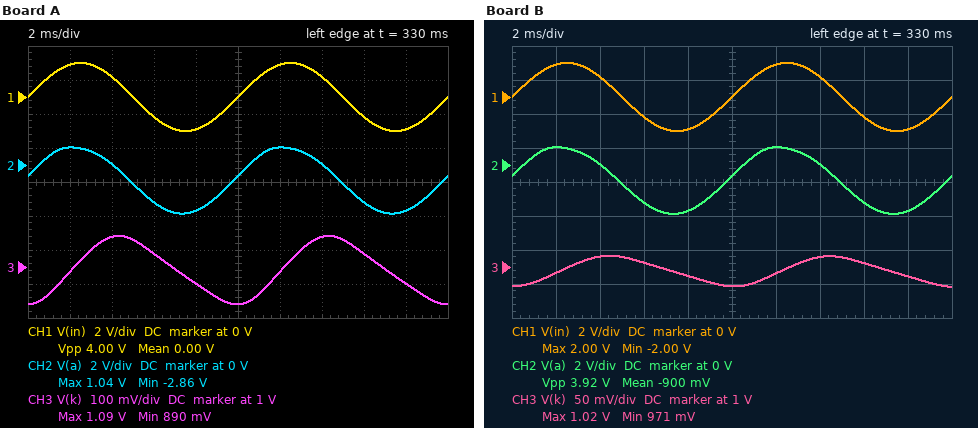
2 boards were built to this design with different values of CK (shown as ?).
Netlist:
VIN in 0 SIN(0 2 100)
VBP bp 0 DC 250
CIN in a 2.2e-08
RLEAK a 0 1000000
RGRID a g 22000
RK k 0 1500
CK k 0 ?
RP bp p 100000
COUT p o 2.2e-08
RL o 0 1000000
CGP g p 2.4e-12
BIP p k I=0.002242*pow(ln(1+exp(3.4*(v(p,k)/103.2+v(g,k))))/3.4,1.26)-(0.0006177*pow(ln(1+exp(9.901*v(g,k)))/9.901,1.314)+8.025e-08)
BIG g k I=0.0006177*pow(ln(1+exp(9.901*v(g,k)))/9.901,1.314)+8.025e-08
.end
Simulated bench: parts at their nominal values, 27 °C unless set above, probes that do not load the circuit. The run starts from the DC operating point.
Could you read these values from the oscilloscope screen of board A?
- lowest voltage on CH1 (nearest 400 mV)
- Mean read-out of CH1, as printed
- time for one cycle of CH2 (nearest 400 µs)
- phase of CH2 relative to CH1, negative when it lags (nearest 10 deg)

-2.0 V
0.00 V
10.0 ms
10 deg
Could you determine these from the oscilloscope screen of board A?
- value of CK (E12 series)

15 µF
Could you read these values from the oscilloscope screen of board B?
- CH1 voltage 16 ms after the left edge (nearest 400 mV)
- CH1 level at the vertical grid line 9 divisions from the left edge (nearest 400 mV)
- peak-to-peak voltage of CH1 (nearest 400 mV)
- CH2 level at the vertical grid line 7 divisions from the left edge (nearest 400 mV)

-1.2 V
-2.0 V
4.0 V
0 V
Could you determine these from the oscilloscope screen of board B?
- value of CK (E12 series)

68 µF
